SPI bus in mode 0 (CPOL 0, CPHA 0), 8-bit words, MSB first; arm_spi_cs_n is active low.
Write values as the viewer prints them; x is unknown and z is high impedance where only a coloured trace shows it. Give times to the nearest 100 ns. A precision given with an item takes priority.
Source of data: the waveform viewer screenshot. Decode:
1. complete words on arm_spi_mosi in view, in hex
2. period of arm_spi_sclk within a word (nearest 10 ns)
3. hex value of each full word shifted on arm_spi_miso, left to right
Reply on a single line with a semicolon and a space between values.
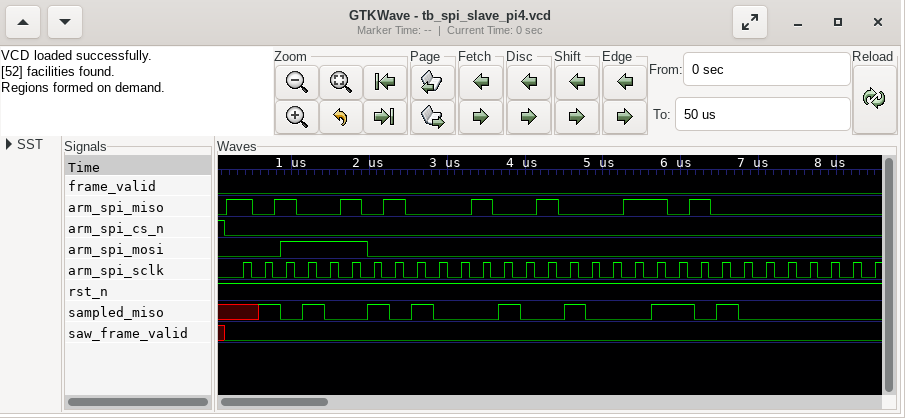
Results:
3C, 00, 00; 280 ns; A5, 12, 34
